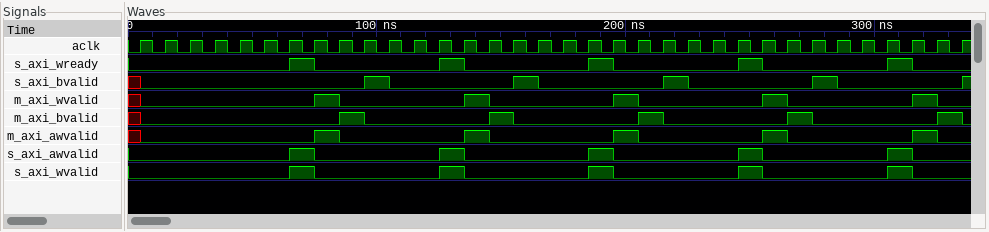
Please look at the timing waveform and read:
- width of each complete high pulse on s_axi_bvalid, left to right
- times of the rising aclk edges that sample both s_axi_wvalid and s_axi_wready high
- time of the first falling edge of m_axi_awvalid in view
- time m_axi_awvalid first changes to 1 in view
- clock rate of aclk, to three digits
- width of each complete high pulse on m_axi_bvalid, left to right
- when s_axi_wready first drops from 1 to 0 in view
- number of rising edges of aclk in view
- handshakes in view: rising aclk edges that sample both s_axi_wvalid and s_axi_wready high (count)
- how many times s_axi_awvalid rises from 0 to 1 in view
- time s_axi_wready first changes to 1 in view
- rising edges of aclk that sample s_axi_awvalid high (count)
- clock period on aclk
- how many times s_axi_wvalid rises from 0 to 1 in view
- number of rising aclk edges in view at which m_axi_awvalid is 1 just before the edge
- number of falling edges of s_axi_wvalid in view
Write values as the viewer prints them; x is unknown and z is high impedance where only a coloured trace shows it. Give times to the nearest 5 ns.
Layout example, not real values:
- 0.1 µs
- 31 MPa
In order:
- 10 ns, 10 ns, 10 ns, 10 ns
- 75 ns, 135 ns, 195 ns, 255 ns, 315 ns
- 85 ns
- 75 ns
- 100 MHz
- 10 ns, 10 ns, 10 ns, 10 ns, 10 ns
- 75 ns
- 34
- 5
- 5
- 65 ns
- 5
- 10 ns
- 5
- 5
- 5
